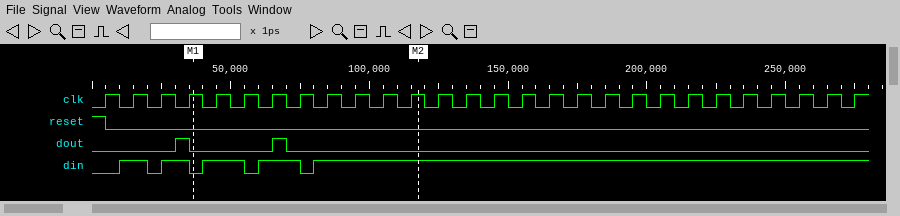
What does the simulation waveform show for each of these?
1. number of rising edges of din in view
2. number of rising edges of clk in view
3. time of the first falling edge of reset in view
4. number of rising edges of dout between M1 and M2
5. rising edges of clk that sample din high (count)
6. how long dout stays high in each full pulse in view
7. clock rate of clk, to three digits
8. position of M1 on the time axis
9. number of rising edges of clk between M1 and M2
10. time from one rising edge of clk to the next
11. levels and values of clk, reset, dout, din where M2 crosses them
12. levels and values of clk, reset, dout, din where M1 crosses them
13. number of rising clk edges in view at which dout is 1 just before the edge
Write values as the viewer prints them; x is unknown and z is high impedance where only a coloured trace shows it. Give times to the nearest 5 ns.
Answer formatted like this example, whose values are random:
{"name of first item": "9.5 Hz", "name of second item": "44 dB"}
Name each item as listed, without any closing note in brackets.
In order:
{"number of rising edges of din in view": "5", "number of rising edges of clk in view": "28", "time of the first falling edge of reset in view": "5 ns", "number of rising edges of dout between M1 and M2": "1", "rising edges of clk that sample din high": "26", "how long dout stays high in each full pulse in view": "5 ns, 5 ns", "clock rate of clk, to three digits": "100 MHz", "position of M1 on the time axis": "35 ns", "number of rising edges of clk between M1 and M2": "8", "time from one rising edge of clk to the next": "10 ns", "levels and values of clk, reset, dout, din where M2 crosses them": "clk=1, reset=0, dout=0, din=1", "levels and values of clk, reset, dout, din where M1 crosses them": "clk=1, reset=0, dout=0, din=0", "number of rising clk edges in view at which dout is 1 just before the edge": "1"}
